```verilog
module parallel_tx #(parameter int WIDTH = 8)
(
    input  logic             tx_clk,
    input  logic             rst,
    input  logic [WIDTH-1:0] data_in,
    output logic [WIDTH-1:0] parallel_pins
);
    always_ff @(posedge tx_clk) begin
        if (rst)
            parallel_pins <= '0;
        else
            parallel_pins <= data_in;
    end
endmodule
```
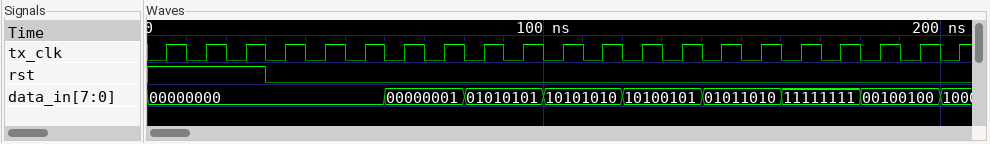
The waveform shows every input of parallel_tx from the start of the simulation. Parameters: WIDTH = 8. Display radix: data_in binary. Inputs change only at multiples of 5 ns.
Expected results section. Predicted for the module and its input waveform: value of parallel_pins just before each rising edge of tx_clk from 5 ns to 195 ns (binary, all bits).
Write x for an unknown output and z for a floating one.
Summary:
x, 00000000, 00000000, 00000000, 00000000, 00000000, 00000000, 00000001, 00000001, 01010101, 01010101, 10101010, 10101010, 10100101, 10100101, 01011010, 01011010, 11111111, 11111111, 00100100
